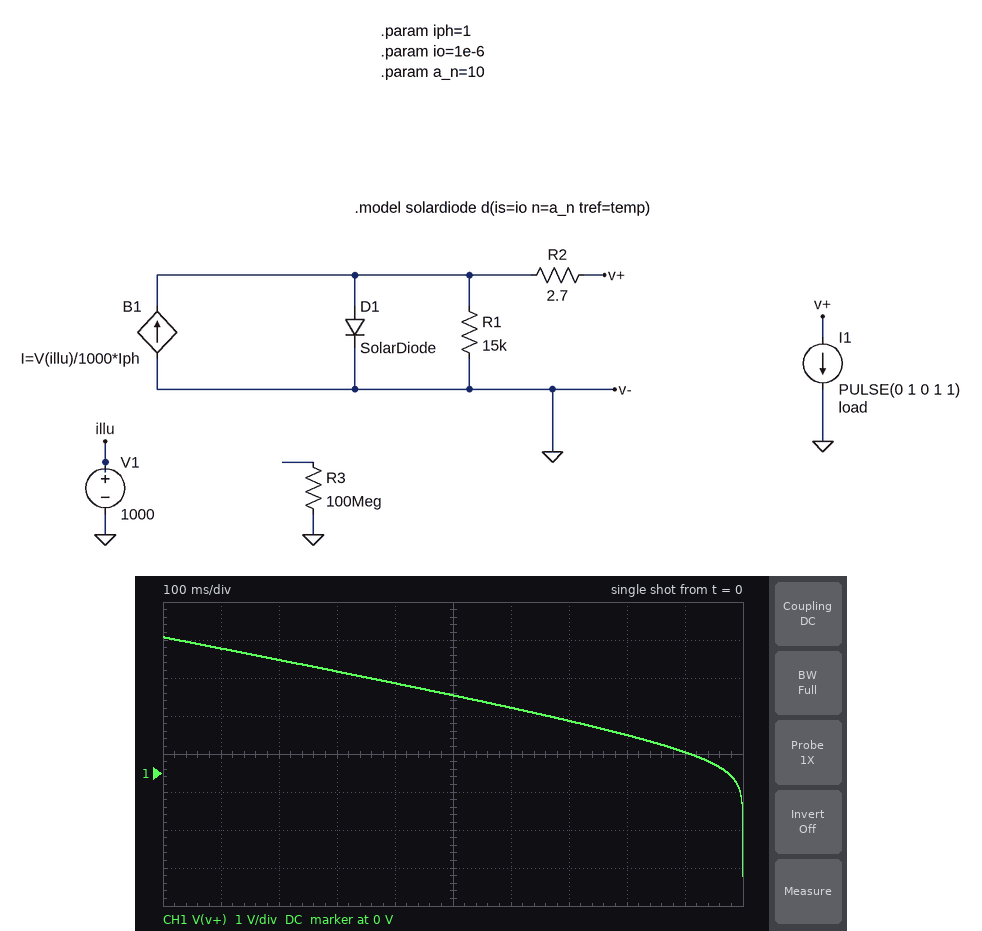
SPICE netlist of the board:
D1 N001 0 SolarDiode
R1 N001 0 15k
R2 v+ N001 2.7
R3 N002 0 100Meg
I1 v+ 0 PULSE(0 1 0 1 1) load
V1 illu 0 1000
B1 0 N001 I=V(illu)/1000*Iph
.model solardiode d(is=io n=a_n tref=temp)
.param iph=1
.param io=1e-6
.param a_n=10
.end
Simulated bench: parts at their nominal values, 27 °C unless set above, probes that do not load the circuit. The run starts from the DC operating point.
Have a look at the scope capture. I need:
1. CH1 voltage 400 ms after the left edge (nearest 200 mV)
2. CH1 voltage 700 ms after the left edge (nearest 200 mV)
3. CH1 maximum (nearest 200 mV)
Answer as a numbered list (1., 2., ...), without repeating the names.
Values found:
1. 2.4 V
2. 1.4 V
3. 3.6 V
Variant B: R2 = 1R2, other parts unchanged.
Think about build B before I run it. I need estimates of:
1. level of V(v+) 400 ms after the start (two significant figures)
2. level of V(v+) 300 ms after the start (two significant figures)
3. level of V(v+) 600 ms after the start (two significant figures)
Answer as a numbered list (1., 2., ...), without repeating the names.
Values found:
1. 3.0 V
2. 3.1 V
3. 2.6 V
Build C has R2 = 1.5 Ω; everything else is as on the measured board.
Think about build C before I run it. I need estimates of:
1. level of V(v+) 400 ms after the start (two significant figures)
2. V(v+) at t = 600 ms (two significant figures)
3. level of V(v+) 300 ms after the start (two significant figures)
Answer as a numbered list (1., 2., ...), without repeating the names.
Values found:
1. 2.8 V
2. 2.4 V
3. 3.0 V
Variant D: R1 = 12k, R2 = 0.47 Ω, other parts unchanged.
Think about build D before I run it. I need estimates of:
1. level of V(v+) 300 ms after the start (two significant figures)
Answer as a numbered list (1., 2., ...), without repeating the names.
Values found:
1. 3.3 V
